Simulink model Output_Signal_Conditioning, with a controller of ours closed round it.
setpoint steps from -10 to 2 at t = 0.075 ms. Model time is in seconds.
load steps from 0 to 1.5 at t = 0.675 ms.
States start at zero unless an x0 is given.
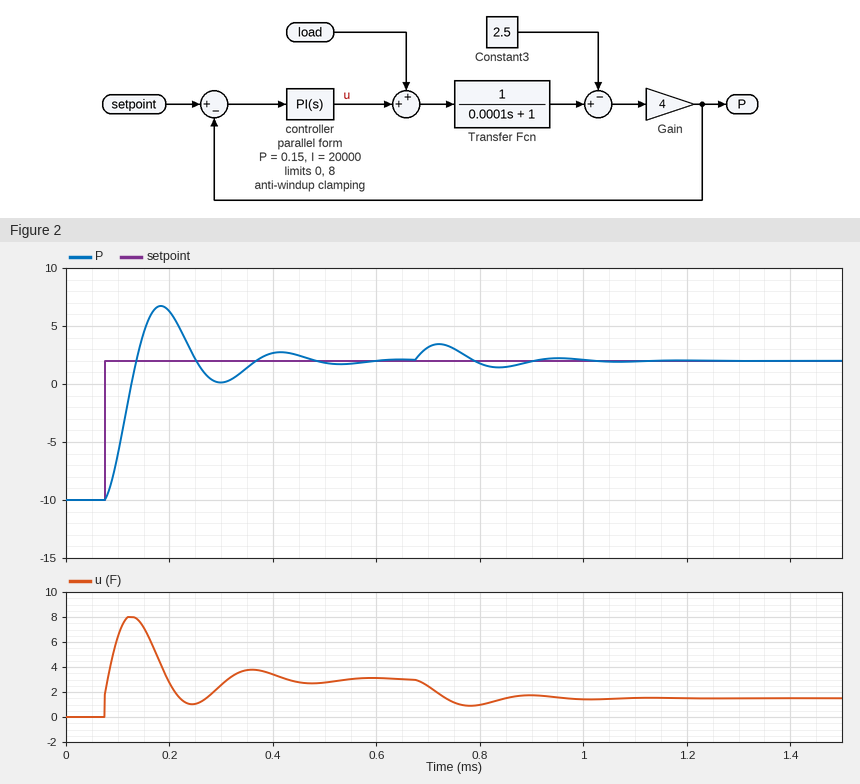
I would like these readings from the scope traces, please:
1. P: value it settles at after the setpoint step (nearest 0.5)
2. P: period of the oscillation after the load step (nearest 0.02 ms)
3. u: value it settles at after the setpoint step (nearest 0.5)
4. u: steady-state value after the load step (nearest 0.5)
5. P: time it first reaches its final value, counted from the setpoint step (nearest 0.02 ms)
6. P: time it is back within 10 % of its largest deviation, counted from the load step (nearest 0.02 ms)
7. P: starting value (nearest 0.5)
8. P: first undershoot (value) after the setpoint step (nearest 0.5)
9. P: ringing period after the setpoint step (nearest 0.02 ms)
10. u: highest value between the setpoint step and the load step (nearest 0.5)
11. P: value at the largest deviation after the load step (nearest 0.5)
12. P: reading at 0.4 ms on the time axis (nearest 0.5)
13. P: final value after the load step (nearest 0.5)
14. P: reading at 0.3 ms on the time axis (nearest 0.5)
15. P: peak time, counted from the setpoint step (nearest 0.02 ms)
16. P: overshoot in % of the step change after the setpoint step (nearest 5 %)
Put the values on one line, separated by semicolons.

2.0; 0.24 ms; 3.0; 1.5; 0.06 ms; 0.32 ms; -10.0; 0.0; 0.24 ms; 8.0; 3.5; 2.5; 2.0; 0.0; 0.10 ms; 40 %
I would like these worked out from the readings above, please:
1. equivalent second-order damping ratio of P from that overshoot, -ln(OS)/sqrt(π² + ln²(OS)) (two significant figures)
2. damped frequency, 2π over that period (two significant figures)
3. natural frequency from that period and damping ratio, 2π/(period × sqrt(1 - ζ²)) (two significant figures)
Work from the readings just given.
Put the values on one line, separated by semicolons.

0.28; 26 rad/ms; 27 rad/ms
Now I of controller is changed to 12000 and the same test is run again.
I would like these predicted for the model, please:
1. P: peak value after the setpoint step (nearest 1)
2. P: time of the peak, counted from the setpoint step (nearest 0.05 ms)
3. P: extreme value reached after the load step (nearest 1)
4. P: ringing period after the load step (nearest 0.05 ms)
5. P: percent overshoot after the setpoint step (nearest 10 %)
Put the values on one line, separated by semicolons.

6; 0.15 ms; 4; 0.30 ms; 30 %
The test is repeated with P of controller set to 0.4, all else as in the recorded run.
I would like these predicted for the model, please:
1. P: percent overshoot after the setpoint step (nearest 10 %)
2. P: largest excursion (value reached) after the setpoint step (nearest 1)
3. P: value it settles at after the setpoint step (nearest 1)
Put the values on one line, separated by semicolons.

20 %; 5; 2
